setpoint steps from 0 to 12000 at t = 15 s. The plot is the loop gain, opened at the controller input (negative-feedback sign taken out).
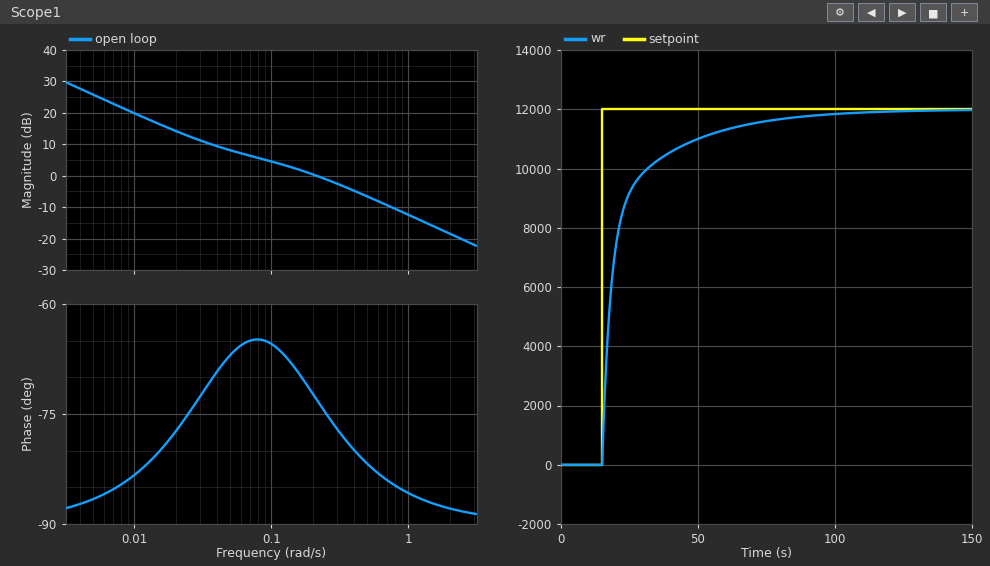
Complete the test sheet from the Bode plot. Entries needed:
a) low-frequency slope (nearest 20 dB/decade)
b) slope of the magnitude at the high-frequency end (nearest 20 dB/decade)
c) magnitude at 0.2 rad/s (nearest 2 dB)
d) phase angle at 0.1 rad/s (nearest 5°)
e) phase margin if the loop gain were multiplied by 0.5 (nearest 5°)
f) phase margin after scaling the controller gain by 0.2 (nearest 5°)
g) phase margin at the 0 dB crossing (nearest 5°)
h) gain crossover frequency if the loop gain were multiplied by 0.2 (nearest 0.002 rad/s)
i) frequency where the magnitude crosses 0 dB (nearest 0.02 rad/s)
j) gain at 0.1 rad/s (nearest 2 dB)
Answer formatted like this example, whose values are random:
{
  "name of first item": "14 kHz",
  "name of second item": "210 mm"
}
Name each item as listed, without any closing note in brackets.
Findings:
{
  "low-frequency slope": "-20 dB/decade",
  "slope of the magnitude at the high-frequency end": "-20 dB/decade",
  "magnitude at 0.2 rad/s": "0 dB",
  "phase angle at 0.1 rad/s": "-65°",
  "phase margin if the loop gain were multiplied by 0.5": "115°",
  "phase margin after scaling the controller gain by 0.2": "105°",
  "phase margin at the 0 dB crossing": "105°",
  "gain crossover frequency if the loop gain were multiplied by 0.2": "0.020 rad/s",
  "frequency where the magnitude crosses 0 dB": "0.22 rad/s",
  "gain at 0.1 rad/s": "4 dB"
}
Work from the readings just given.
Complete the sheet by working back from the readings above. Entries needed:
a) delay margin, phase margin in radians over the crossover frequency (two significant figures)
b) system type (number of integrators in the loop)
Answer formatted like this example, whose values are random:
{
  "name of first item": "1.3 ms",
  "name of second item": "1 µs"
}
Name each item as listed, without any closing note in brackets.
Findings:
{
  "delay margin, phase margin in radians over the crossover frequency": "8.3 s",
  "system type": "1"
}
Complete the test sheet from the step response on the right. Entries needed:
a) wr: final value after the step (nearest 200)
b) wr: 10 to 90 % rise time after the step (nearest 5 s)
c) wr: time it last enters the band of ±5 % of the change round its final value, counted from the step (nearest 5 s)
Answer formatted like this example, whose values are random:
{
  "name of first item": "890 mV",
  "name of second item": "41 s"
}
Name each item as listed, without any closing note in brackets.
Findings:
{
  "wr: final value after the step": "12000",
  "wr: 10 to 90 % rise time after the step": "30 s",
  "wr: time it last enters the band of ±5 % of the change round its final value, counted from the step": "50 s"
}
